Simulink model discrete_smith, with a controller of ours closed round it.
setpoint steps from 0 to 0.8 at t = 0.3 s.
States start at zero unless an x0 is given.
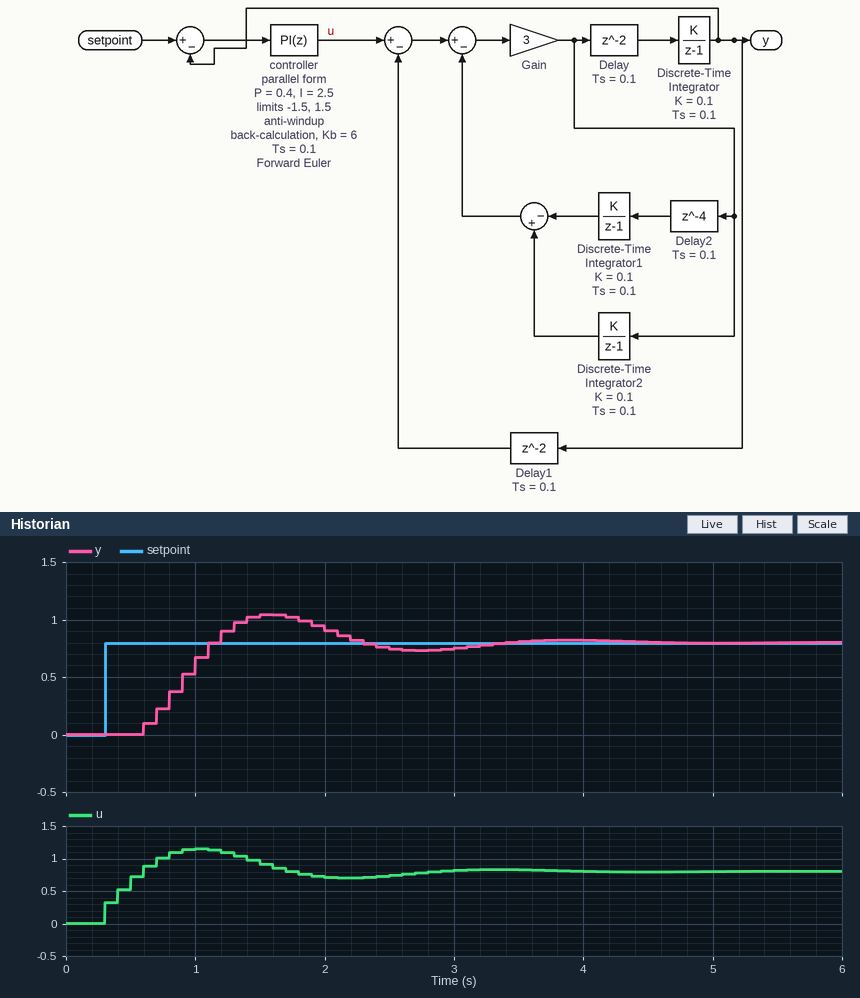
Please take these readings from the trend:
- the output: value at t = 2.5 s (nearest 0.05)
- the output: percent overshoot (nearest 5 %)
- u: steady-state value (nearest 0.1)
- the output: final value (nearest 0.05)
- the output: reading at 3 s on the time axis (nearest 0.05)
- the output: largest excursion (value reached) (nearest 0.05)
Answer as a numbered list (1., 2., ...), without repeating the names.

1. 0.75
2. 30 %
3. 0.8
4. 0.80
5. 0.75
6. 1.05
